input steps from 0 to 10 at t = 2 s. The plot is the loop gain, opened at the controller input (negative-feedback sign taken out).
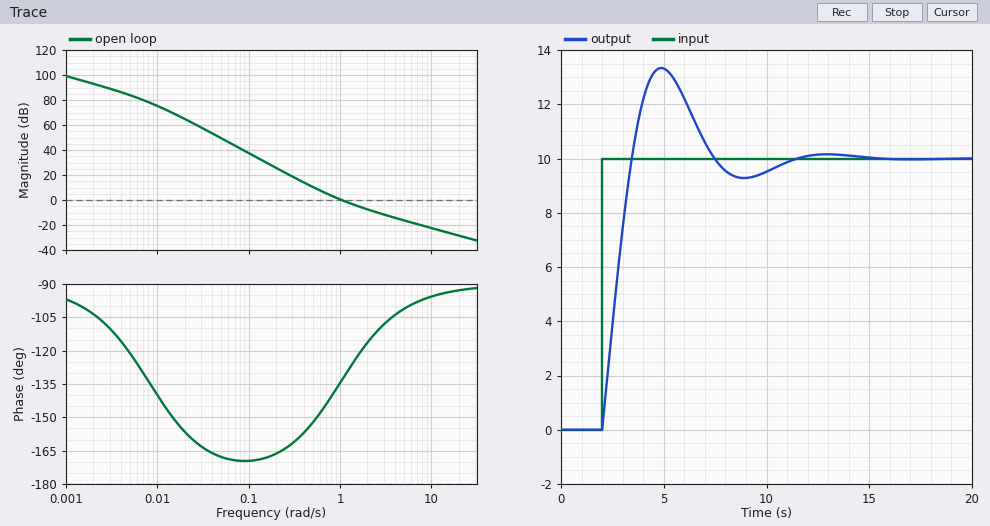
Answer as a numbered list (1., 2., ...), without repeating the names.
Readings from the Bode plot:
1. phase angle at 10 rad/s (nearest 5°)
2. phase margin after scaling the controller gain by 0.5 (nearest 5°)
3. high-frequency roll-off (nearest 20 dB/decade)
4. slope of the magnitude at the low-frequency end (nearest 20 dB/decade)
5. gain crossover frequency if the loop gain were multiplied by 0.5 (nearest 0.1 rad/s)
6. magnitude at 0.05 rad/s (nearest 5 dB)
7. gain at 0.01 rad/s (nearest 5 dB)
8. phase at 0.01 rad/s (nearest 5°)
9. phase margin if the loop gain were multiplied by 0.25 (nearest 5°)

1. -95°
2. 35°
3. -20 dB/decade
4. -20 dB/decade
5. 0.7 rad/s
6. 50 dB
7. 75 dB
8. -140°
9. 25°
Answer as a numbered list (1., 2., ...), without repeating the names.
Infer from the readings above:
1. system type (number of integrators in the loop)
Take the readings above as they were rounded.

1. 1
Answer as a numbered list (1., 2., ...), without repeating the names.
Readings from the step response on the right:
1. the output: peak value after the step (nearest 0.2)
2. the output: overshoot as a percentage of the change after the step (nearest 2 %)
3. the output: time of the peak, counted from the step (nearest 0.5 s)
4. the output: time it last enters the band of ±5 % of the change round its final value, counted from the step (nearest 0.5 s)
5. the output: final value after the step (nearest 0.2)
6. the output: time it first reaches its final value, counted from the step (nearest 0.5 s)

1. 13.4
2. 34 %
3. 3.0 s
4. 8.0 s
5. 10.0
6. 1.5 s
